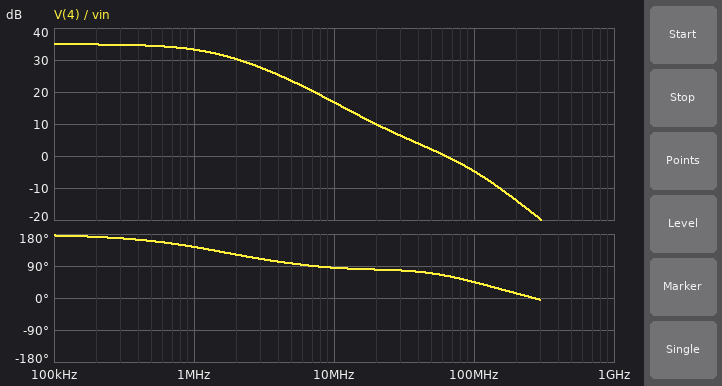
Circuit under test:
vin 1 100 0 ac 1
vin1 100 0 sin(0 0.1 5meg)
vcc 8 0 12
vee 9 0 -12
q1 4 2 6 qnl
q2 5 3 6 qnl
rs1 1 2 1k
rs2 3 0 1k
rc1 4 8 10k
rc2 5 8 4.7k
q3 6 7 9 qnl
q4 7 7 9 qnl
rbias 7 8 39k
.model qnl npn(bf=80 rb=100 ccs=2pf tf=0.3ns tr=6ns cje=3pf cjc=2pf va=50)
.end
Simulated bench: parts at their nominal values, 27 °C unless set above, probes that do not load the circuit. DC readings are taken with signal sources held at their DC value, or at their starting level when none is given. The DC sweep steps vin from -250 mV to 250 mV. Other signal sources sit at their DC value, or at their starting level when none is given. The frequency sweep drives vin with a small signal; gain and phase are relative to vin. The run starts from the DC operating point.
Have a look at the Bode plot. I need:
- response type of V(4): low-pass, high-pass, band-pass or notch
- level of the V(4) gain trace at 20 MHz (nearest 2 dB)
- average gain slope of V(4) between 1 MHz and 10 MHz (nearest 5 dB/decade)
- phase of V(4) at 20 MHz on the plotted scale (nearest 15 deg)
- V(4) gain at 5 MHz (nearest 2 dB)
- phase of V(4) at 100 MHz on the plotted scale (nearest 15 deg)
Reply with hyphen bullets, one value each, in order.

- low-pass
- 10 dB
- -15 dB/decade
- 75 deg
- 24 dB
- 45 deg
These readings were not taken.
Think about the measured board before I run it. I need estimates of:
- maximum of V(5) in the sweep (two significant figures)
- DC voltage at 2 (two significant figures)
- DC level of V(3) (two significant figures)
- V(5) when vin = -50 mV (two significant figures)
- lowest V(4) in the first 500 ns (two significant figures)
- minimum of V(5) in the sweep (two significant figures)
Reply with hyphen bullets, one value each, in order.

- 12 V
- -3.7 mV
- -3.7 mV
- 9.2 V
- 6.6 V
- 8.7 V
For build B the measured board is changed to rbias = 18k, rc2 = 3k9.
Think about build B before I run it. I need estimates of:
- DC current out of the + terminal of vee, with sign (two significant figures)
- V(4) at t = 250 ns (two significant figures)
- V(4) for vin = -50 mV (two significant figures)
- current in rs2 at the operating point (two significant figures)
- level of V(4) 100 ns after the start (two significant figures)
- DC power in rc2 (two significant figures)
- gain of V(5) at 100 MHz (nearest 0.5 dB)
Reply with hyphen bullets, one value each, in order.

- -2.8 mA
- 4.3 V
- 9.2 V
- 8.3 µA
- 2.3 V
- 2.4 mW
- -10.0 dB
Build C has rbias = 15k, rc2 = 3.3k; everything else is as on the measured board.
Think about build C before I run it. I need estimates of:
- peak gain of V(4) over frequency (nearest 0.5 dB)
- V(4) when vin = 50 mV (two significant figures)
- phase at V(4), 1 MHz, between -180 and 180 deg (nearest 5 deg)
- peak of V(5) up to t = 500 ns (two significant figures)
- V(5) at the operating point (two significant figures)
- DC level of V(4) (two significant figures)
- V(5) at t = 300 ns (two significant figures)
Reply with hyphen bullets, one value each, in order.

- 41.0 dB
- -630 mV
- 125 deg
- 9.9 V
- 8.9 V
- 3.4 V
- 9.6 V
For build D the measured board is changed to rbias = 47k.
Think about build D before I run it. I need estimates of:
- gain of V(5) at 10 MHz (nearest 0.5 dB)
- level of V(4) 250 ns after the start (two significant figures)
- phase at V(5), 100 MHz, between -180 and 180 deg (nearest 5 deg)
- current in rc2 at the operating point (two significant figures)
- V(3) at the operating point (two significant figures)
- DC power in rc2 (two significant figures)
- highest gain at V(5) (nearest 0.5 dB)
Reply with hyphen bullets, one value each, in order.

- 14.0 dB
- 8.8 V
- -155 deg
- 290 µA
- -3.0 mV
- 400 µW
- 27.0 dB
